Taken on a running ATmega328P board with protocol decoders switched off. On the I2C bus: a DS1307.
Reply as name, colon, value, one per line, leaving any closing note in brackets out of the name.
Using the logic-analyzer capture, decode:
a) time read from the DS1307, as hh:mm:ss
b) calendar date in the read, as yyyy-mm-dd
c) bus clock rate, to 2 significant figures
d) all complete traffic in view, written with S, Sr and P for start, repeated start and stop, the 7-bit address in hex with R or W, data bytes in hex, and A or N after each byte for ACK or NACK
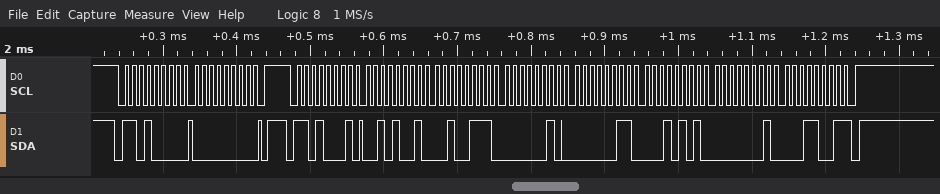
time read from the DS1307, as hh:mm:ss: 02:27:29
calendar date in the read, as yyyy-mm-dd: 2019-01-15
bus clock rate, to 2 significant figures: 100 kHz
all complete traffic in view, written with S, Sr and P for start, repeated start and stop, the 7-bit address in hex with R or W, data bytes in hex, and A or N after each byte for ACK or NACK: S 68W A 00 A P S 68R A 29 A 27 A 02 A 03 A 15 A 01 A 19 N P
